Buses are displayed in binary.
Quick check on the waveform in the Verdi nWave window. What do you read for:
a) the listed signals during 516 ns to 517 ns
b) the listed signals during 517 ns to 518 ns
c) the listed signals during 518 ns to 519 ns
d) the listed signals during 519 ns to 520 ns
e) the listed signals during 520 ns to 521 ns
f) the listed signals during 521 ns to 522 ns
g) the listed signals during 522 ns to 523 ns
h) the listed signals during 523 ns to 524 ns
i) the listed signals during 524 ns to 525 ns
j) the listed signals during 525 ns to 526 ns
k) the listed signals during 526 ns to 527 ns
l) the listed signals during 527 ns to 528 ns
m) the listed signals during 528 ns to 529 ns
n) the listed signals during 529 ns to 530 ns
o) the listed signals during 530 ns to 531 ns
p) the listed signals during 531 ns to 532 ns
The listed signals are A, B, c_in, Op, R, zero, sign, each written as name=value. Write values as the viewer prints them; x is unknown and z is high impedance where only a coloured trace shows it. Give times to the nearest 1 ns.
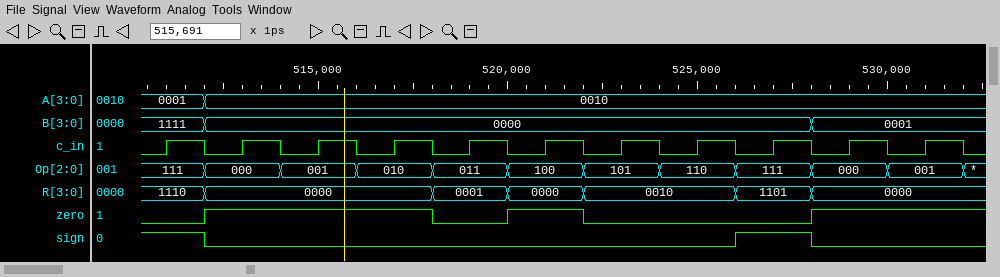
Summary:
A=0010, B=0000, c_in=0, Op=010, R=0000, zero=1, sign=0
A=0010, B=0000, c_in=1, Op=010, R=0000, zero=1, sign=0
A=0010, B=0000, c_in=0, Op=011, R=0001, zero=0, sign=0
A=0010, B=0000, c_in=1, Op=011, R=0001, zero=0, sign=0
A=0010, B=0000, c_in=0, Op=100, R=0000, zero=1, sign=0
A=0010, B=0000, c_in=1, Op=100, R=0000, zero=1, sign=0
A=0010, B=0000, c_in=0, Op=101, R=0010, zero=0, sign=0
A=0010, B=0000, c_in=1, Op=101, R=0010, zero=0, sign=0
A=0010, B=0000, c_in=0, Op=110, R=0010, zero=0, sign=0
A=0010, B=0000, c_in=1, Op=110, R=0010, zero=0, sign=0
A=0010, B=0000, c_in=0, Op=111, R=1101, zero=0, sign=1
A=0010, B=0000, c_in=1, Op=111, R=1101, zero=0, sign=1
A=0010, B=0001, c_in=0, Op=000, R=0000, zero=1, sign=0
A=0010, B=0001, c_in=1, Op=000, R=0000, zero=1, sign=0
A=0010, B=0001, c_in=0, Op=001, R=0000, zero=1, sign=0
A=0010, B=0001, c_in=1, Op=001, R=0000, zero=1, sign=0
